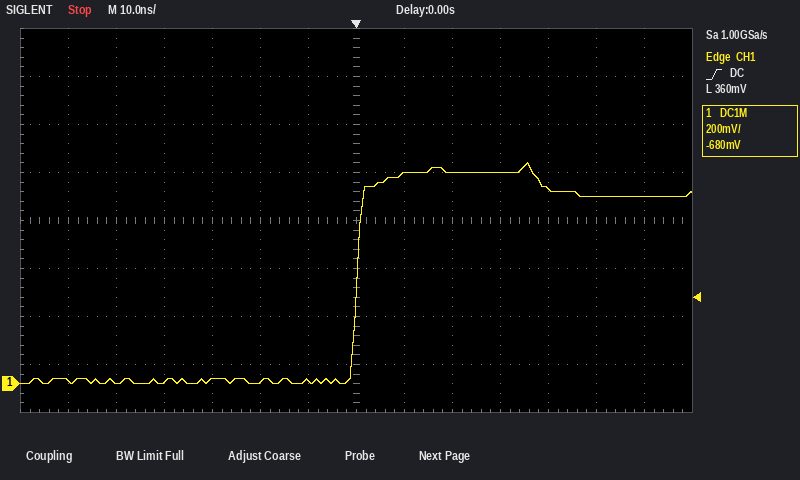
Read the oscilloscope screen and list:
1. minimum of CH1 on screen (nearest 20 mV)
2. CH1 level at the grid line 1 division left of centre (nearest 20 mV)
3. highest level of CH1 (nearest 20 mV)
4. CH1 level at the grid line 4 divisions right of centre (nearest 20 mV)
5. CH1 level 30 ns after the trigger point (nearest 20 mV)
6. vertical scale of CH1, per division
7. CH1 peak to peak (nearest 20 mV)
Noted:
0 mV
20 mV
920 mV
820 mV
880 mV
200 mV
920 mV
